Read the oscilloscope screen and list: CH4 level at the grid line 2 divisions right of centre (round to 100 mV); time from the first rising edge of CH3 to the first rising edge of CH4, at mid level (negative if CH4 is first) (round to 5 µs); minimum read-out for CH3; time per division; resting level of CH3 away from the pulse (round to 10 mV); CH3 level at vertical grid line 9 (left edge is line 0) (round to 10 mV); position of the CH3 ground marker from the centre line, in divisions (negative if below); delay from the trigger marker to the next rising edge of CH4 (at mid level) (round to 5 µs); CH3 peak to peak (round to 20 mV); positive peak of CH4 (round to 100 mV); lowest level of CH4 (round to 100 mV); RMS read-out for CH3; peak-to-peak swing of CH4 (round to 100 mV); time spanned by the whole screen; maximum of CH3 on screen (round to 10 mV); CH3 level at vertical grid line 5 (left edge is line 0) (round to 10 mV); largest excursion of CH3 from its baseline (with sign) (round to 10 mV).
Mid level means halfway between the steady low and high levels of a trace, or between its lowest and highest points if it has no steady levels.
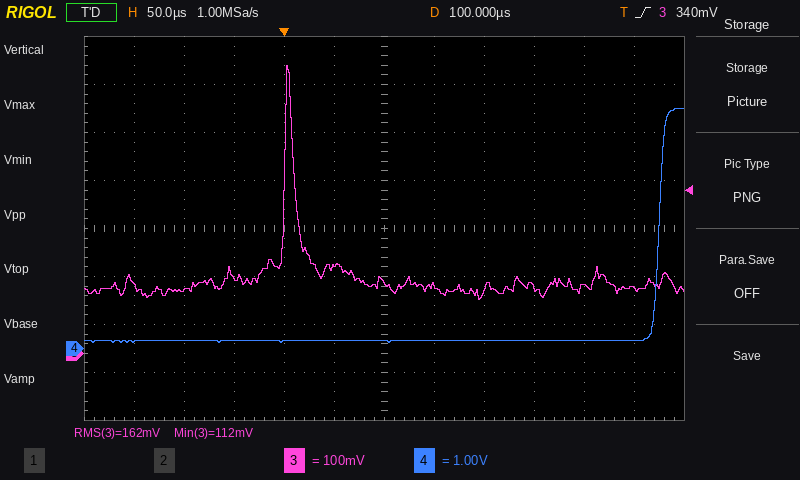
200 mV
+375 µs
112 mV
50 µs
140 mV
140 mV
-2.6 div
375 µs
480 mV
5.0 V
100 mV
162 mV
4.9 V
600 µs
600 mV
180 mV
+460 mV
